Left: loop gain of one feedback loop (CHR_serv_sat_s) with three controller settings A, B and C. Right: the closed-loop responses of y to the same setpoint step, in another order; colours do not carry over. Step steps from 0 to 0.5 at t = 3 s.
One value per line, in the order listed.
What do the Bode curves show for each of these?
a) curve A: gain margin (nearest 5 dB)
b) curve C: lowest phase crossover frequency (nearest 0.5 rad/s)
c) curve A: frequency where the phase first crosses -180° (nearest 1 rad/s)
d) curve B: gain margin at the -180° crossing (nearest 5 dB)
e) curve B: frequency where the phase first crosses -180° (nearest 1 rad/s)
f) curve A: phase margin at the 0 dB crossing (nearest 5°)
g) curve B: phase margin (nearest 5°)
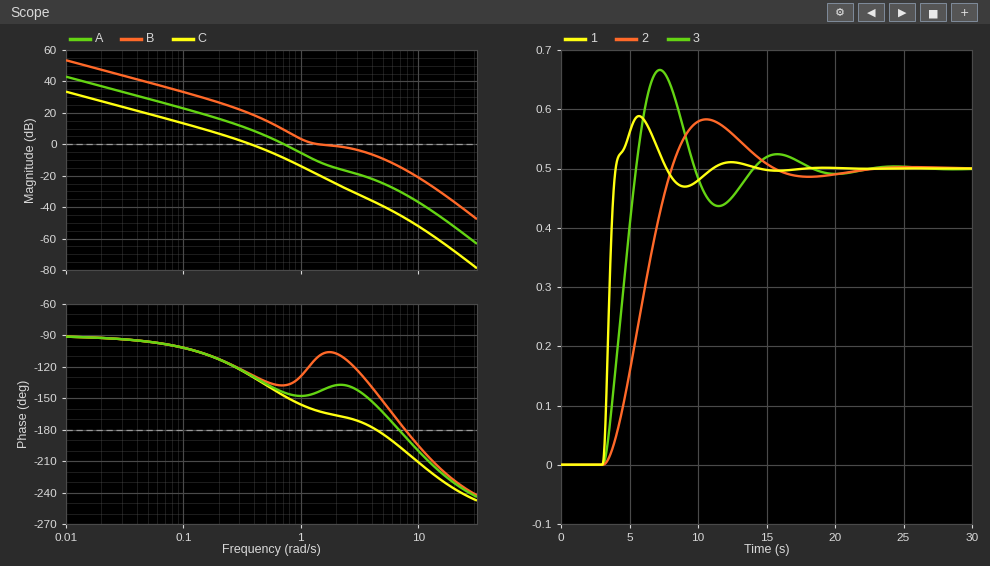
30 dB
4.5 rad/s
7 rad/s
15 dB
8 rad/s
35°
70°
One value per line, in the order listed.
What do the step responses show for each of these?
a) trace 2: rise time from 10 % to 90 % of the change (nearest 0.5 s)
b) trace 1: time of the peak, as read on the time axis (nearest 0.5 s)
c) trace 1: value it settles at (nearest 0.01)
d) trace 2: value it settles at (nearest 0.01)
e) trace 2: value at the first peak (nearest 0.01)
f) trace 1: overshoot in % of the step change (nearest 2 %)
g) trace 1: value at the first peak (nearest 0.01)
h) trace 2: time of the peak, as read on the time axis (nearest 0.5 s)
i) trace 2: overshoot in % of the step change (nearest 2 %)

3.5 s
5.5 s
0.50
0.50
0.58
18 %
0.59
10.5 s
16 %
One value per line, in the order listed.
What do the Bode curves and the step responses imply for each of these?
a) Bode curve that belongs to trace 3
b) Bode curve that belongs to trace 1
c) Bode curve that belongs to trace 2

A
B
C
